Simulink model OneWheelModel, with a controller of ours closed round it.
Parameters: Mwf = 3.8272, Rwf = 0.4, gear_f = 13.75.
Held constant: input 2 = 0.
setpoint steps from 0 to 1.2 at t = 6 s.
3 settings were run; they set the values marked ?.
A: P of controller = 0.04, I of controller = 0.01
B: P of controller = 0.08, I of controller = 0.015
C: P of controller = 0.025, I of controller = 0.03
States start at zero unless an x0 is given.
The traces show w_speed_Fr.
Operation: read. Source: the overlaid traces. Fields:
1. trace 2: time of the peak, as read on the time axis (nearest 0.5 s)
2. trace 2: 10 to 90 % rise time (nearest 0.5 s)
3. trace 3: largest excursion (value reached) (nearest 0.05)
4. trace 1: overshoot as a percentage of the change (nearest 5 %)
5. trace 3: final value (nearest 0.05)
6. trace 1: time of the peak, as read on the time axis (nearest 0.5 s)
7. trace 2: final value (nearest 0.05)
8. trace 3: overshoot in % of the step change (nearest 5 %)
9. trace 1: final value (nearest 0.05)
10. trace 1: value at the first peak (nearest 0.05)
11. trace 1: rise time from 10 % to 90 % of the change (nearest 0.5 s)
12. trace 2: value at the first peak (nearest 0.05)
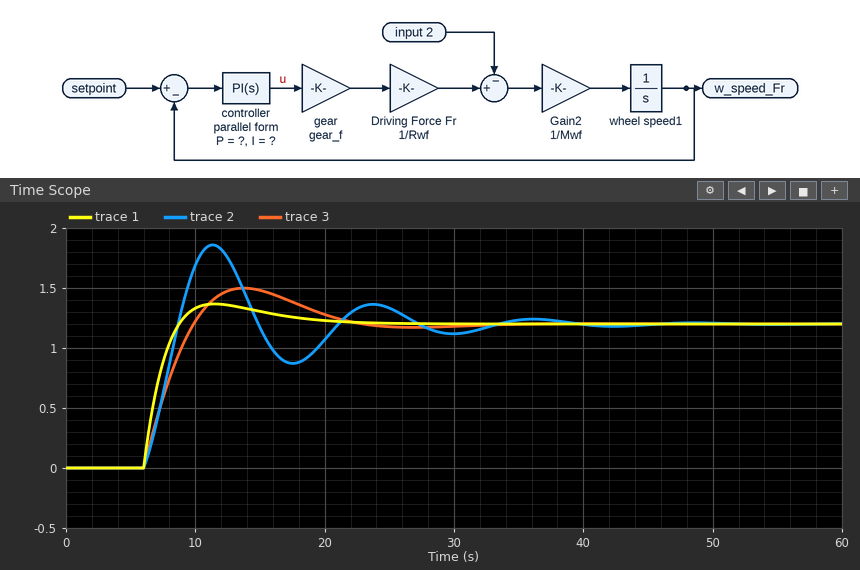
11.5 s
2.0 s
1.50
15 %
1.20
11.5 s
1.20
25 %
1.20
1.35
2.0 s
1.85
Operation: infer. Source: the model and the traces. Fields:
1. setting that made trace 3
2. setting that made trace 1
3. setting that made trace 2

A
B
C
